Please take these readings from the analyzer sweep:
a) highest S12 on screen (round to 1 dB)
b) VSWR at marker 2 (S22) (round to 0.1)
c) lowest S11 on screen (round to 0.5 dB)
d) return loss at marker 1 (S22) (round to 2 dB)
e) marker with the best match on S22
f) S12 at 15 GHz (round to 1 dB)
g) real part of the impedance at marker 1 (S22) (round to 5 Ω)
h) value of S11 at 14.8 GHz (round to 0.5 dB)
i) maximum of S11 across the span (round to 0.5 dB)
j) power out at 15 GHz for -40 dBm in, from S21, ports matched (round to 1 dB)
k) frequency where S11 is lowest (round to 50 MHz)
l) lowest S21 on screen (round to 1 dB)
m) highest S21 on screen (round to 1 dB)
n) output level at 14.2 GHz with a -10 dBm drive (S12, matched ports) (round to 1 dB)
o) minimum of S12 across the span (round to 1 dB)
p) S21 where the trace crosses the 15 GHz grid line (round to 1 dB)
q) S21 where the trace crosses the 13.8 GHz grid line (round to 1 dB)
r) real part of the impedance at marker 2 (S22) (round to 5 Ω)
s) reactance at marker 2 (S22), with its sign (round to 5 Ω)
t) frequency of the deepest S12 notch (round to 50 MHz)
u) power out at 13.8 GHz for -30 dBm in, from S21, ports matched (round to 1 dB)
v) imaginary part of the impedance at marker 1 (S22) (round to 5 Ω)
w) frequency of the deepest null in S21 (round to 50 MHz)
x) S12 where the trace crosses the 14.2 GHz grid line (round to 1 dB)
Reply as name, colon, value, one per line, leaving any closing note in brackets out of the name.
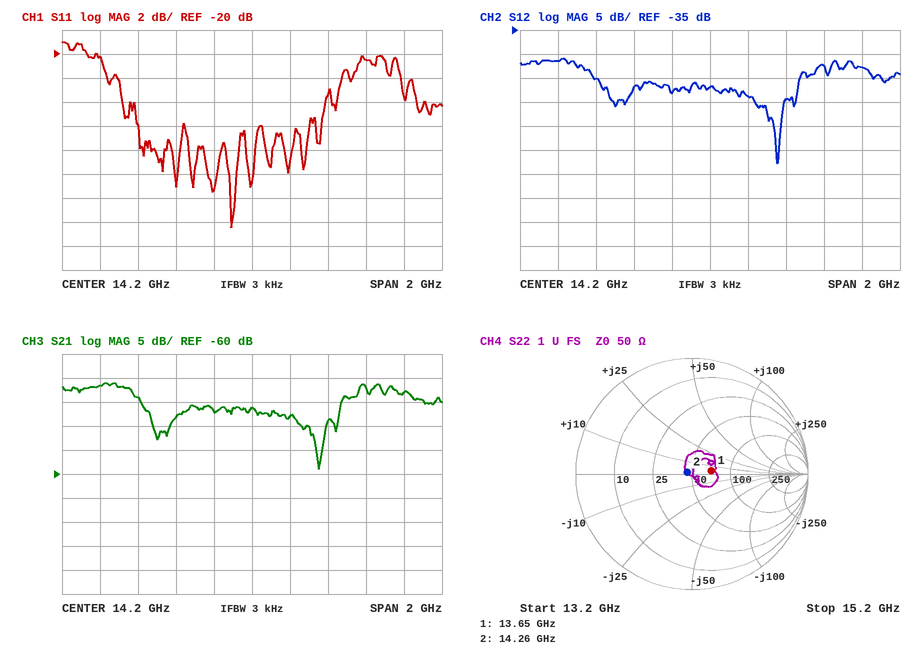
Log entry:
highest S12 on screen: -41 dB
VSWR at marker 2 (S22): 1.1
lowest S11 on screen: -34.5 dB
return loss at marker 1 (S22): 16 dB
marker with the best match on S22: marker 2
S12 at 15 GHz: -43 dB
real part of the impedance at marker 1 (S22): 70 Ω
value of S11 at 14.8 GHz: -20.5 dB
maximum of S11 across the span: -19.0 dB
power out at 15 GHz for -40 dBm in, from S21, ports matched: -83 dBm
frequency where S11 is lowest: 14.10 GHz
lowest S21 on screen: -59 dB
highest S21 on screen: -41 dB
output level at 14.2 GHz with a -10 dBm drive (S12, matched ports): -57 dBm
minimum of S12 across the span: -63 dB
S21 where the trace crosses the 15 GHz grid line: -43 dB
S21 where the trace crosses the 13.8 GHz grid line: -48 dB
real part of the impedance at marker 2 (S22): 45 Ω
reactance at marker 2 (S22), with its sign: 0 Ω
frequency of the deepest S12 notch: 14.55 GHz
power out at 13.8 GHz for -30 dBm in, from S21, ports matched: -78 dBm
imaginary part of the impedance at marker 1 (S22): +5 Ω
frequency of the deepest null in S21: 14.55 GHz
S12 where the trace crosses the 14.2 GHz grid line: -47 dB
